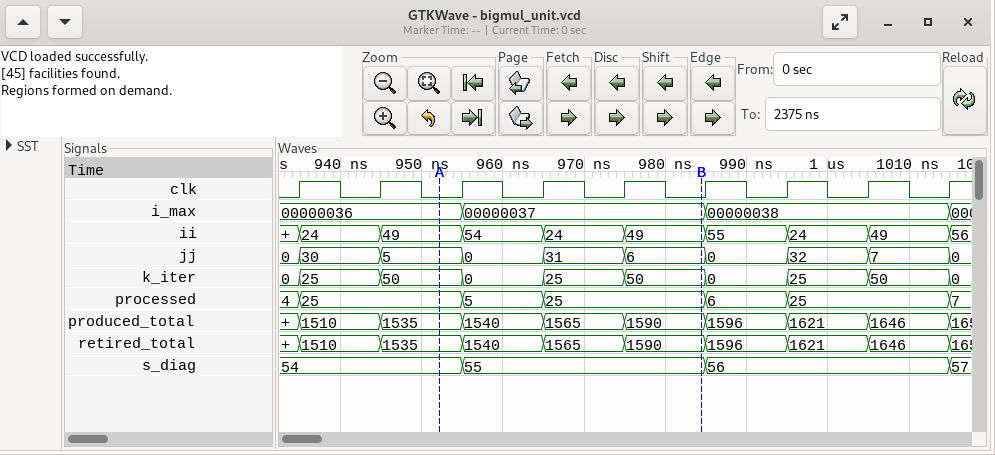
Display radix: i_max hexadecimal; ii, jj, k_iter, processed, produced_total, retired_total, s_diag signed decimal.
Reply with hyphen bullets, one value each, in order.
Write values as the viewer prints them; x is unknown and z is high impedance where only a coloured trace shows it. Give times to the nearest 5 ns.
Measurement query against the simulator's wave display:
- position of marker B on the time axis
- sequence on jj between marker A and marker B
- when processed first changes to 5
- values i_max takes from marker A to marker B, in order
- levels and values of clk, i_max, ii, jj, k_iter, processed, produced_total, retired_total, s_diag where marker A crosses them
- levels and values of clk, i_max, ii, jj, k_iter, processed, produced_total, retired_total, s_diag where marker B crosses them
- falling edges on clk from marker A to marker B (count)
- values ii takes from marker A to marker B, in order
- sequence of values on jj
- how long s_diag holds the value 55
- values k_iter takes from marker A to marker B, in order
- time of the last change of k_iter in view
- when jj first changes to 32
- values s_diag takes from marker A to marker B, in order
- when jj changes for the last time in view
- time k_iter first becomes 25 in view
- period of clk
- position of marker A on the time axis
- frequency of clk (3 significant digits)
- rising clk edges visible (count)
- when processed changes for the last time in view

- 985 ns
- 5, 0, 31, 6
- 955 ns
- 00000036, 00000037
- clk=0, i_max=00000036, ii=49, jj=5, k_iter=50, processed=25, produced_total=1535, retired_total=1535, s_diag=54
- clk=0, i_max=00000037, ii=49, jj=6, k_iter=50, processed=25, produced_total=1590, retired_total=1590, s_diag=55
- 3
- 49, 54, 24, 49
- 0, 30, 5, 0, 31, 6, 0, 32, 7, 0
- 30 ns
- 50, 0, 25, 50
- 1015 ns
- 995 ns
- 54, 55
- 1015 ns
- 935 ns
- 10 ns
- 950 ns
- 100 MHz
- 9
- 1015 ns
